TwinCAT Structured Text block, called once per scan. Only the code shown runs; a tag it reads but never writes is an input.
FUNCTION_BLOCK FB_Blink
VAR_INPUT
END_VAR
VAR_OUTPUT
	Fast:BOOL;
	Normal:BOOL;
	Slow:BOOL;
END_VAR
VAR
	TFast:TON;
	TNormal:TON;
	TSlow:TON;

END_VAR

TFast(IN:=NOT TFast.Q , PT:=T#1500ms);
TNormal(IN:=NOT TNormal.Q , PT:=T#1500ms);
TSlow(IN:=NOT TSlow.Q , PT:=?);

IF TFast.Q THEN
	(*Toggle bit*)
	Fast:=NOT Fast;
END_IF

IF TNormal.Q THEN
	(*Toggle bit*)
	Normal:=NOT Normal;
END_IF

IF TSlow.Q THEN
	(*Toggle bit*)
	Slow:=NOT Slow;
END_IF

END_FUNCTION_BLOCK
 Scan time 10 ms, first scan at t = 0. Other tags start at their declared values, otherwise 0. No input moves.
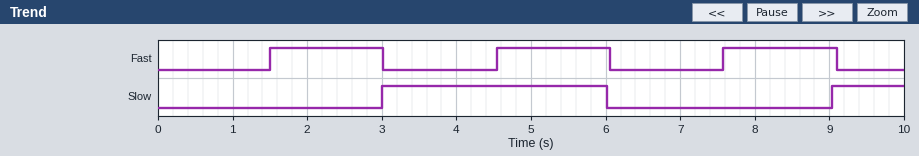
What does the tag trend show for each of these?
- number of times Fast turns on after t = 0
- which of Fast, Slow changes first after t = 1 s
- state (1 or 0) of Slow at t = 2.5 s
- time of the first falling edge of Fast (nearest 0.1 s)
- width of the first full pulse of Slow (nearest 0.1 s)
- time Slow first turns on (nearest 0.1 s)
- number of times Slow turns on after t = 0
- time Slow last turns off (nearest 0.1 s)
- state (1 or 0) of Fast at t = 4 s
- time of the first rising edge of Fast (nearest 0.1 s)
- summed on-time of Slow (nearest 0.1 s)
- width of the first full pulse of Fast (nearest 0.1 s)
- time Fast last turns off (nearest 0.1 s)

3
Fast
0
3.0 s
3.0 s
3.0 s
2
6.0 s
0
1.5 s
4.0 s
1.5 s
9.1 s
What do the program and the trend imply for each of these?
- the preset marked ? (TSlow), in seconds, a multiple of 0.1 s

3.0 s
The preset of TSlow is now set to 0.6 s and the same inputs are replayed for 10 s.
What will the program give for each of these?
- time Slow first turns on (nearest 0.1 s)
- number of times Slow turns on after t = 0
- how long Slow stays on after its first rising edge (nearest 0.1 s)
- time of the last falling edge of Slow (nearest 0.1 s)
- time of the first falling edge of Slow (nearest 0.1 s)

0.6 s
8
0.6 s
9.9 s
1.2 s
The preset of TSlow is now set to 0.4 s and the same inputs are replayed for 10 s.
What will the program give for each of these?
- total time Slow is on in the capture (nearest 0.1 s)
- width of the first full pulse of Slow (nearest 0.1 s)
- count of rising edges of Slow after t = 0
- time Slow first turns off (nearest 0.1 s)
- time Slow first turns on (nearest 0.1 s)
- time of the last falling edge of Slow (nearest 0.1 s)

5.0 s
0.4 s
12
0.8 s
0.4 s
9.2 s
